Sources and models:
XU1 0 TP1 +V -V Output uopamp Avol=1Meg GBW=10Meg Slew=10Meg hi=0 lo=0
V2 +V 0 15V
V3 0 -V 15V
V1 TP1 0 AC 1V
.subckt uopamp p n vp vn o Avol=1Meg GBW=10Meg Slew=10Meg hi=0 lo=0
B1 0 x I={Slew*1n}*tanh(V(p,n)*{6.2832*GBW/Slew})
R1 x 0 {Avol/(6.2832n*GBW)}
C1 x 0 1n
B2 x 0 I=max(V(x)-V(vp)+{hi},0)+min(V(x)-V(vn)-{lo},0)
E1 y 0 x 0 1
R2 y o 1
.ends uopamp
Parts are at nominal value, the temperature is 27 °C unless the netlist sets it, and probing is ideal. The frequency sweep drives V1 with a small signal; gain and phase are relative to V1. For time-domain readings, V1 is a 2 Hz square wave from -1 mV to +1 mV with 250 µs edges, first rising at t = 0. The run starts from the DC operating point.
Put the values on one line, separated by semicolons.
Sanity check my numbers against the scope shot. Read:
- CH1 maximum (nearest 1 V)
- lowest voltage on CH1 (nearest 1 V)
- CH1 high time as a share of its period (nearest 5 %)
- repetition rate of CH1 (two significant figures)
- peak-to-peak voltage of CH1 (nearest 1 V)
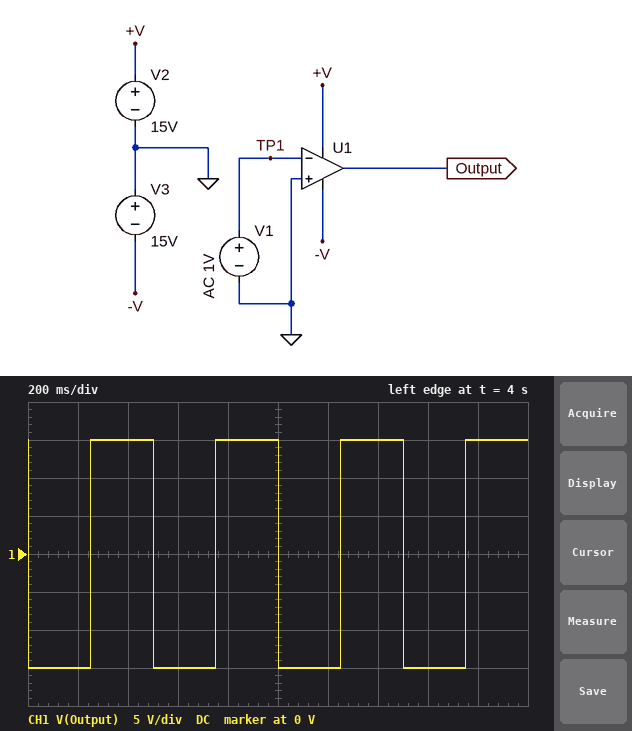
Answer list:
15 V; -15 V; 50 %; 2.0 Hz; 30 V
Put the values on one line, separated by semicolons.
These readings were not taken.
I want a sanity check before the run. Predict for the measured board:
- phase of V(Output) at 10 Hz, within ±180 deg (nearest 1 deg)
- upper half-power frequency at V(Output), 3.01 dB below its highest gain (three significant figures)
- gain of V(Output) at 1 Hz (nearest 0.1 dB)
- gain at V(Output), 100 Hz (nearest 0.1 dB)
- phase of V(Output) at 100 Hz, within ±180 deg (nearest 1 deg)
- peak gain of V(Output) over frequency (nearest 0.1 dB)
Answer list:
135 deg; 10.0 Hz; 120.0 dB; 100.0 dB; 96 deg; 120.0 dB
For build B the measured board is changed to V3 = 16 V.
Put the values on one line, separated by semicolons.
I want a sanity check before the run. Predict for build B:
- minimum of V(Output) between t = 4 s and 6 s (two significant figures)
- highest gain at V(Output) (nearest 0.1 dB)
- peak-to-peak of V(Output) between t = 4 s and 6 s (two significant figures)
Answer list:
-16 V; 120.0 dB; 31 V
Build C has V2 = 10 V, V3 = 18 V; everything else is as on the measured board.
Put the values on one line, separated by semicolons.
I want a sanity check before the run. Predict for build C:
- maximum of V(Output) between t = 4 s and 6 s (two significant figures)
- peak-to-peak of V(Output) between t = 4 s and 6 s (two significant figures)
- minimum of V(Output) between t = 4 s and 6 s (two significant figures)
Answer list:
10 V; 28 V; -18 V
